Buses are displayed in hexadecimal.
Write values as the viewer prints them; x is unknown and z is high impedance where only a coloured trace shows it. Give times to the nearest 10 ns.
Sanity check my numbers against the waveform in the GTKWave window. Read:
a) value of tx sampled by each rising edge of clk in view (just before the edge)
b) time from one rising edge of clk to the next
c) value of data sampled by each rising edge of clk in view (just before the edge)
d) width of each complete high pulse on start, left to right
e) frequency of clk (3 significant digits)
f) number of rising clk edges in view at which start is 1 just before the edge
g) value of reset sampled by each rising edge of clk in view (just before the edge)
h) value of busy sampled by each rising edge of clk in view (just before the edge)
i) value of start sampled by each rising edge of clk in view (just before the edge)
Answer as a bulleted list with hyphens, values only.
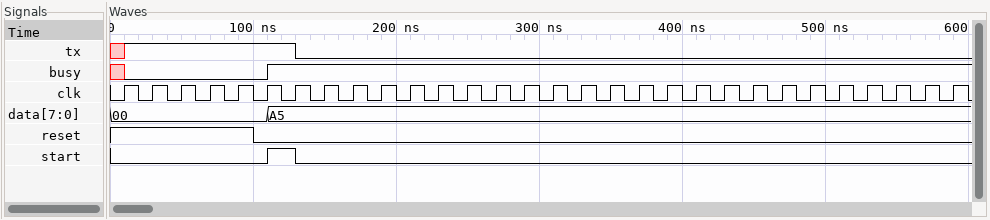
- x 1 1 1 1 1 1 0 0 0 0 0 0 0 0 0 0 0 0 0 0 0 0 0 0 0 0 0 0 0
- 20 ns
- 00, 00, 00, 00, 00, 00, A5, A5, A5, A5, A5, A5, A5, A5, A5, A5, A5, A5, A5, A5, A5, A5, A5, A5, A5, A5, A5, A5, A5, A5
- 20 ns
- 50.0 MHz
- 1
- 1 1 1 1 1 0 0 0 0 0 0 0 0 0 0 0 0 0 0 0 0 0 0 0 0 0 0 0 0 0
- x 0 0 0 0 0 1 1 1 1 1 1 1 1 1 1 1 1 1 1 1 1 1 1 1 1 1 1 1 1
- 0 0 0 0 0 0 1 0 0 0 0 0 0 0 0 0 0 0 0 0 0 0 0 0 0 0 0 0 0 0
